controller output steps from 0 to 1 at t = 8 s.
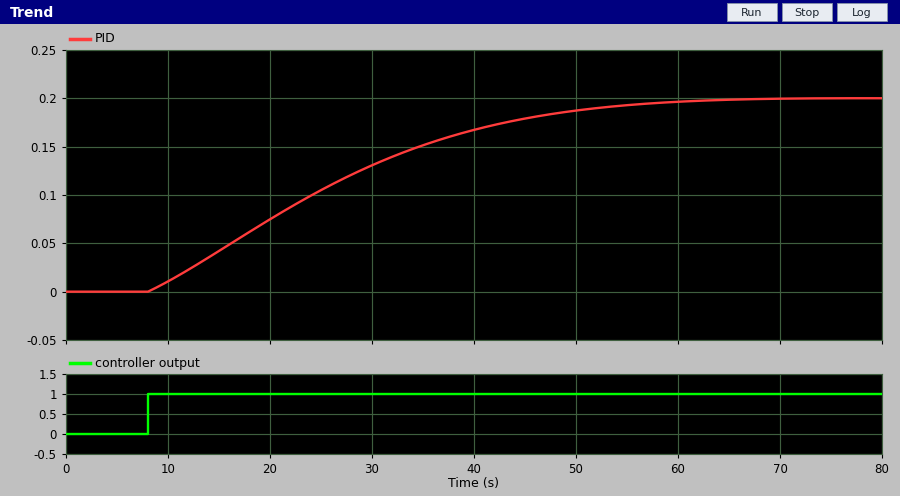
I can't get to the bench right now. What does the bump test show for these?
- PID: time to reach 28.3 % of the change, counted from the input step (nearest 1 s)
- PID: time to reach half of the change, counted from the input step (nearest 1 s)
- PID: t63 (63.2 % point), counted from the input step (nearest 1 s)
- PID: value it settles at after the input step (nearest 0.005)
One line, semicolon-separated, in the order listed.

9 s; 16 s; 21 s; 0.200
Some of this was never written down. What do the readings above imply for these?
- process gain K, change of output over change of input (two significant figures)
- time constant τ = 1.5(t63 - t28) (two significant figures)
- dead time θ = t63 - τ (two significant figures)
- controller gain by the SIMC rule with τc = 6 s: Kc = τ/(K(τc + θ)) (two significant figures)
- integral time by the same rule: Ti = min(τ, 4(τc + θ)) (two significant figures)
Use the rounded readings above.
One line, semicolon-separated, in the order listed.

0.20; 18 s; 3.0 s; 10; 18 s
